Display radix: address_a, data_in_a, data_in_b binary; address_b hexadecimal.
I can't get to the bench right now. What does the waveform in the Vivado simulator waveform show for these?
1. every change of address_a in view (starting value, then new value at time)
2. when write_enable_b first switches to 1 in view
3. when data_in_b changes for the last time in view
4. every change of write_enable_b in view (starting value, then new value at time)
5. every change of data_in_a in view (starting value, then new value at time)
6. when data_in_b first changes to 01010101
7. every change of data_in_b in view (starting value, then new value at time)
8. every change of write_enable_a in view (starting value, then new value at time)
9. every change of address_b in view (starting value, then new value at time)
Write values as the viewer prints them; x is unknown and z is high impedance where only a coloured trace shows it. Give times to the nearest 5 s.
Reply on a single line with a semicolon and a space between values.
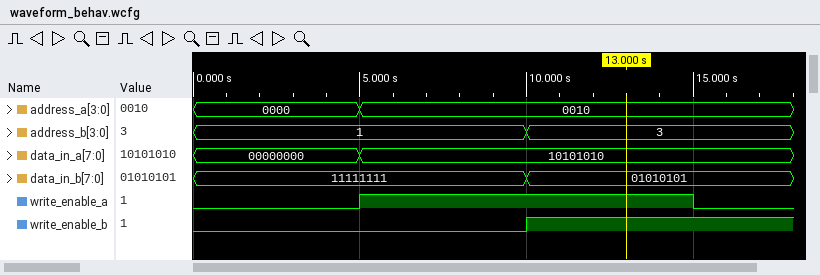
0000, 0010 at 5 s; 10 s; 10 s; 0, 1 at 10 s; 00000000, 10101010 at 5 s; 10 s; 11111111, 01010101 at 10 s; 0, 1 at 5 s, 0 at 15 s; 1, 3 at 10 s
